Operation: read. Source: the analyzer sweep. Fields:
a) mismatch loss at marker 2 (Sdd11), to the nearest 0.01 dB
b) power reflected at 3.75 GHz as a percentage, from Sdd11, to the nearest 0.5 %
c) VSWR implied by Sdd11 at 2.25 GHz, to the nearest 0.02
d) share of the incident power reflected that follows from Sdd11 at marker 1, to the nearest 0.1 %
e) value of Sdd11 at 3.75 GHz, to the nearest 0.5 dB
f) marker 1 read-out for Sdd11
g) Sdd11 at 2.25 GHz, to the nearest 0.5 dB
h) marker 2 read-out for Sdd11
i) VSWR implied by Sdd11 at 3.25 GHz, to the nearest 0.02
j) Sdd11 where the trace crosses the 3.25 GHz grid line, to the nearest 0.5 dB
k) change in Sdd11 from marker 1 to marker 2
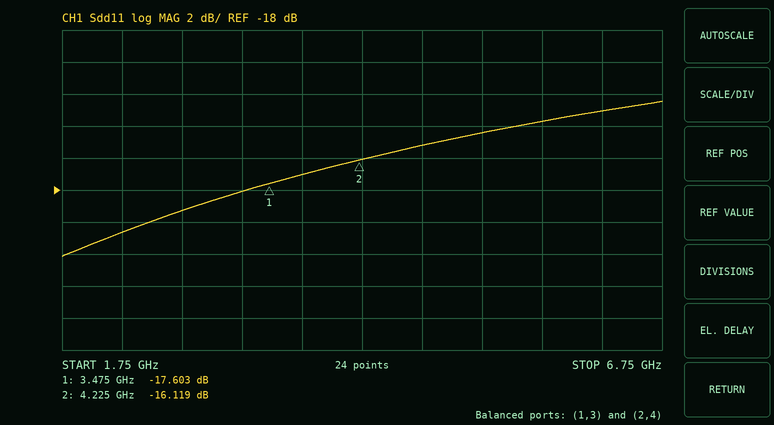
0.11 dB
2.0 %
1.20
1.7 %
-17.0 dB
-17.603 dB
-20.5 dB
-16.119 dB
1.28
-18.0 dB
1.484 dB
